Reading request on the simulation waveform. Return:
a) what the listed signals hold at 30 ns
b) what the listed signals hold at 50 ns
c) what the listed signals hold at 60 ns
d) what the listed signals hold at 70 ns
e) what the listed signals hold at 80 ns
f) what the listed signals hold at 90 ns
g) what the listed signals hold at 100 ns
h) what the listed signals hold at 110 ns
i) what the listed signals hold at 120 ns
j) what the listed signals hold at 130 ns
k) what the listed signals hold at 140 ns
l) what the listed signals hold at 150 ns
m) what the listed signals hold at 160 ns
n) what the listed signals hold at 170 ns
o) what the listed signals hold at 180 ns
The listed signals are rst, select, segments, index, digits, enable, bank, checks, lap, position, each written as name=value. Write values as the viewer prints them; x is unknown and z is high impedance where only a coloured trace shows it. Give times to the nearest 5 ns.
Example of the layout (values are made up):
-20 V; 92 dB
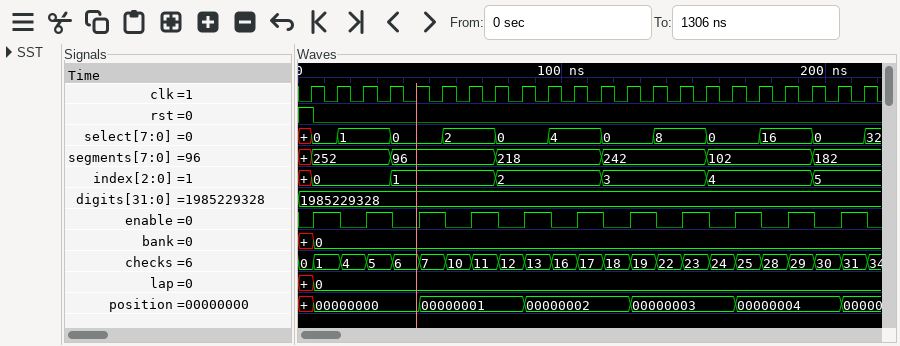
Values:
rst=0, select=1, segments=252, index=0, digits=1985229328, enable=1, bank=0, checks=5, lap=0, position=00000000; rst=0, select=0, segments=96, index=1, digits=1985229328, enable=1, bank=0, checks=7, lap=0, position=00000001; rst=0, select=2, segments=96, index=1, digits=1985229328, enable=0, bank=0, checks=10, lap=0, position=00000001; rst=0, select=2, segments=96, index=1, digits=1985229328, enable=1, bank=0, checks=11, lap=0, position=00000001; rst=0, select=0, segments=218, index=2, digits=1985229328, enable=0, bank=0, checks=12, lap=0, position=00000001; rst=0, select=0, segments=218, index=2, digits=1985229328, enable=1, bank=0, checks=13, lap=0, position=00000002; rst=0, select=4, segments=218, index=2, digits=1985229328, enable=0, bank=0, checks=16, lap=0, position=00000002; rst=0, select=4, segments=218, index=2, digits=1985229328, enable=1, bank=0, checks=17, lap=0, position=00000002; rst=0, select=0, segments=242, index=3, digits=1985229328, enable=0, bank=0, checks=18, lap=0, position=00000002; rst=0, select=0, segments=242, index=3, digits=1985229328, enable=1, bank=0, checks=19, lap=0, position=00000003; rst=0, select=8, segments=242, index=3, digits=1985229328, enable=0, bank=0, checks=22, lap=0, position=00000003; rst=0, select=8, segments=242, index=3, digits=1985229328, enable=1, bank=0, checks=23, lap=0, position=00000003; rst=0, select=0, segments=102, index=4, digits=1985229328, enable=0, bank=0, checks=24, lap=0, position=00000003; rst=0, select=0, segments=102, index=4, digits=1985229328, enable=1, bank=0, checks=25, lap=0, position=00000004; rst=0, select=16, segments=102, index=4, digits=1985229328, enable=0, bank=0, checks=28, lap=0, position=00000004
